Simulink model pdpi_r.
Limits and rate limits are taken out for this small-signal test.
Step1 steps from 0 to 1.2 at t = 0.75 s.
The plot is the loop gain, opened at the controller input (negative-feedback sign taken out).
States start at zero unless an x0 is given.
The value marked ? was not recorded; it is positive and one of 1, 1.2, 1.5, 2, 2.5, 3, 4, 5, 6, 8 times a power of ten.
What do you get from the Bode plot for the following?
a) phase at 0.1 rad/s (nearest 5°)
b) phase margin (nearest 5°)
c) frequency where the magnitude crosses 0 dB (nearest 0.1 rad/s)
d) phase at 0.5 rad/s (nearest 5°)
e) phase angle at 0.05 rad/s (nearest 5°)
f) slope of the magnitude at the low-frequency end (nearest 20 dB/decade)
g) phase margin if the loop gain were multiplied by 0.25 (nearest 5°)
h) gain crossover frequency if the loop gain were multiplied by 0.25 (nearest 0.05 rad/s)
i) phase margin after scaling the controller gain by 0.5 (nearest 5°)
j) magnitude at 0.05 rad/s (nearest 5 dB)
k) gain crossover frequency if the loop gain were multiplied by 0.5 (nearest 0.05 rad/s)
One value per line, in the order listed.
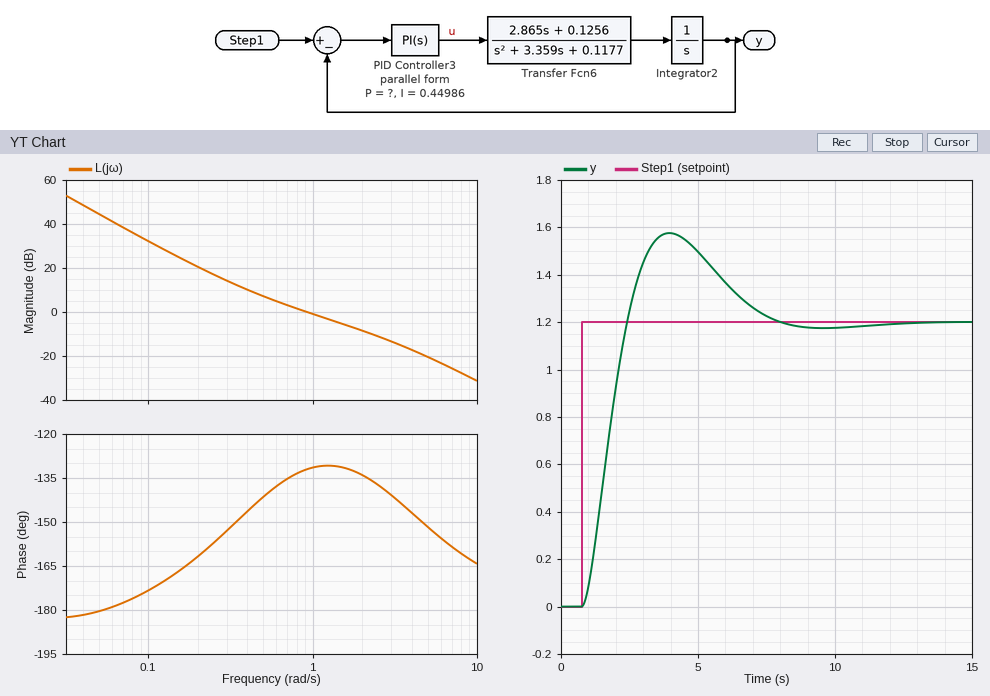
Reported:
-175°
50°
0.9 rad/s
-140°
-180°
-40 dB/decade
30°
0.35 rad/s
40°
45 dB
0.55 rad/s
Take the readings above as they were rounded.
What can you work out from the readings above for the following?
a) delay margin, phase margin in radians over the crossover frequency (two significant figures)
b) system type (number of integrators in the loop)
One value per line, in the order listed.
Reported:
0.97 s
2
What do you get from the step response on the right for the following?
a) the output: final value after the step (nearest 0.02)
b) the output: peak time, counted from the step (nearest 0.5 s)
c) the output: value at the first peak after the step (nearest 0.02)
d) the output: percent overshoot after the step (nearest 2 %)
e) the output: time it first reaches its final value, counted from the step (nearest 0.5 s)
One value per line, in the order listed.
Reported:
1.20
3.0 s
1.58
32 %
1.5 s
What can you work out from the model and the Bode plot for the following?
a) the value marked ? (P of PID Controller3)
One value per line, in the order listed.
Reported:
1
